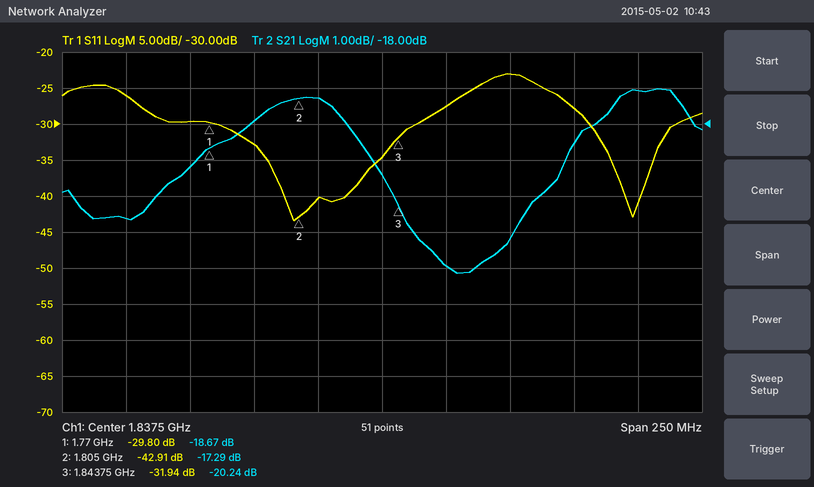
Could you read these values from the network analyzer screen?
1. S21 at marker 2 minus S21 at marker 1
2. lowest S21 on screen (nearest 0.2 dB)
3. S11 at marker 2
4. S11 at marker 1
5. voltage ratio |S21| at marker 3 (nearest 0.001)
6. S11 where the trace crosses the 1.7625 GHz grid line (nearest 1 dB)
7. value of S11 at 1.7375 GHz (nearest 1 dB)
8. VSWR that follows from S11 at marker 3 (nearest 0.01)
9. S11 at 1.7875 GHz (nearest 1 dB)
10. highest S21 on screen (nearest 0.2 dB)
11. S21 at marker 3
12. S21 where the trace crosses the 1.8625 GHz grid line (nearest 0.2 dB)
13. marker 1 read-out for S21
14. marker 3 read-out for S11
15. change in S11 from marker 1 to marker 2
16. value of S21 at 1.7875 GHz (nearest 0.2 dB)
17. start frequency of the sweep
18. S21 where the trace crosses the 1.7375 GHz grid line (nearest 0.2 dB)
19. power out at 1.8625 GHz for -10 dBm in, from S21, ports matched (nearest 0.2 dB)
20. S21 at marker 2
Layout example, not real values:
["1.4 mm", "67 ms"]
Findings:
["1.38 dB", "-22.2 dB", "-42.91 dB", "-29.80 dB", "0.097", "-30 dB", "-26 dB", "1.05", "-33 dB", "-17.0 dB", "-20.24 dB", "-22.0 dB", "-18.67 dB", "-31.94 dB", "-13.11 dB", "-18.0 dB", "1.7125 GHz", "-20.6 dB", "-32.0 dBm", "-17.29 dB"]
